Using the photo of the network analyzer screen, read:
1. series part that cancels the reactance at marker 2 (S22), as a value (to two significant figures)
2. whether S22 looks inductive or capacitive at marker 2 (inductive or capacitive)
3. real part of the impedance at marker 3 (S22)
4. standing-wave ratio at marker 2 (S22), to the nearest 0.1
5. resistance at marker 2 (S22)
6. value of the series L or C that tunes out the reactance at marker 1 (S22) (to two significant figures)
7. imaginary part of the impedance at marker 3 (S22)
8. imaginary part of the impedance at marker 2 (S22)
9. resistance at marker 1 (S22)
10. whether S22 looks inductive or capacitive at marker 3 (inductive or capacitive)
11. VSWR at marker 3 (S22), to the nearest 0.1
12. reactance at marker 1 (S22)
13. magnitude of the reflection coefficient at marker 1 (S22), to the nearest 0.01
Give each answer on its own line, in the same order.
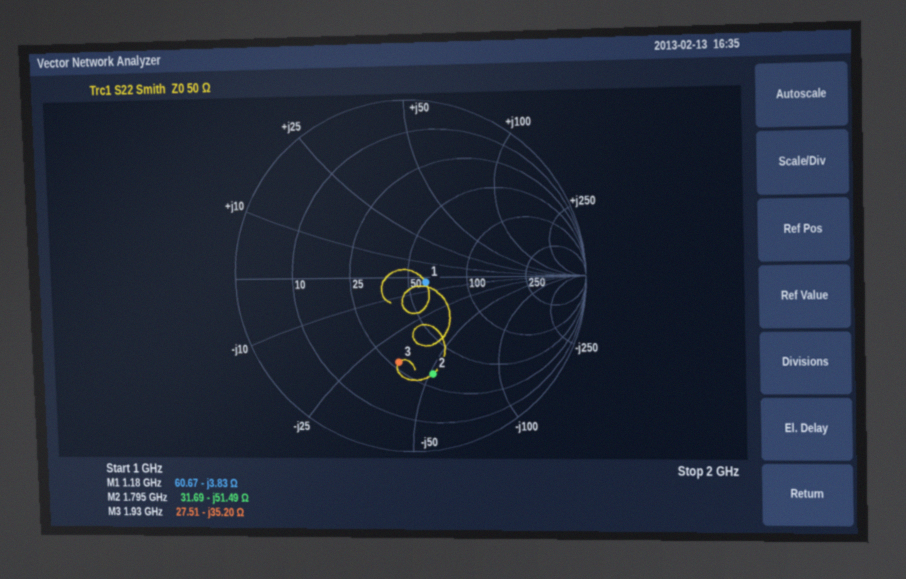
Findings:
4.6 nH
capacitive
27.51 Ω
3.6
31.69 Ω
520 pH
-35.20 Ω
-51.49 Ω
60.67 Ω
capacitive
2.9
-3.83 Ω
0.10
